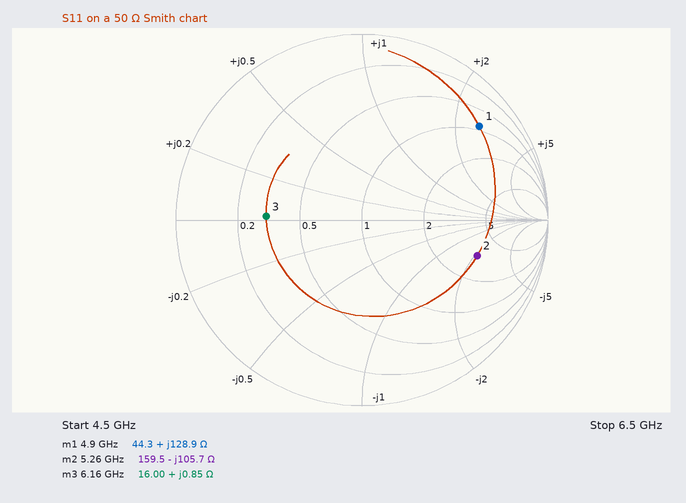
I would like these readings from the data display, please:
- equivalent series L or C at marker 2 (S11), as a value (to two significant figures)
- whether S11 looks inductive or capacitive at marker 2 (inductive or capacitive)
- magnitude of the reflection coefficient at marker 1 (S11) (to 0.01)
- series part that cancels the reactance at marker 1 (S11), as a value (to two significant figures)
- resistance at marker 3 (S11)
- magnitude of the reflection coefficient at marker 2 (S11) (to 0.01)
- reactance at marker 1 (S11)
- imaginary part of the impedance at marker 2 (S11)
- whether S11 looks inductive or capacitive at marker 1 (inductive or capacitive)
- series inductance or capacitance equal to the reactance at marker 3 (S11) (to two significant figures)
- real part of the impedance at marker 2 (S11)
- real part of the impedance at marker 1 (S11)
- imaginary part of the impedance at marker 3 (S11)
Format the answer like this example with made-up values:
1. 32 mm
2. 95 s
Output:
1. 290 fF
2. capacitive
3. 0.81
4. 250 fF
5. 16.00 Ω
6. 0.65
7. +128.9 Ω
8. -105.7 Ω
9. inductive
10. 22 pH
11. 159.5 Ω
12. 44.3 Ω
13. +0.85 Ω
